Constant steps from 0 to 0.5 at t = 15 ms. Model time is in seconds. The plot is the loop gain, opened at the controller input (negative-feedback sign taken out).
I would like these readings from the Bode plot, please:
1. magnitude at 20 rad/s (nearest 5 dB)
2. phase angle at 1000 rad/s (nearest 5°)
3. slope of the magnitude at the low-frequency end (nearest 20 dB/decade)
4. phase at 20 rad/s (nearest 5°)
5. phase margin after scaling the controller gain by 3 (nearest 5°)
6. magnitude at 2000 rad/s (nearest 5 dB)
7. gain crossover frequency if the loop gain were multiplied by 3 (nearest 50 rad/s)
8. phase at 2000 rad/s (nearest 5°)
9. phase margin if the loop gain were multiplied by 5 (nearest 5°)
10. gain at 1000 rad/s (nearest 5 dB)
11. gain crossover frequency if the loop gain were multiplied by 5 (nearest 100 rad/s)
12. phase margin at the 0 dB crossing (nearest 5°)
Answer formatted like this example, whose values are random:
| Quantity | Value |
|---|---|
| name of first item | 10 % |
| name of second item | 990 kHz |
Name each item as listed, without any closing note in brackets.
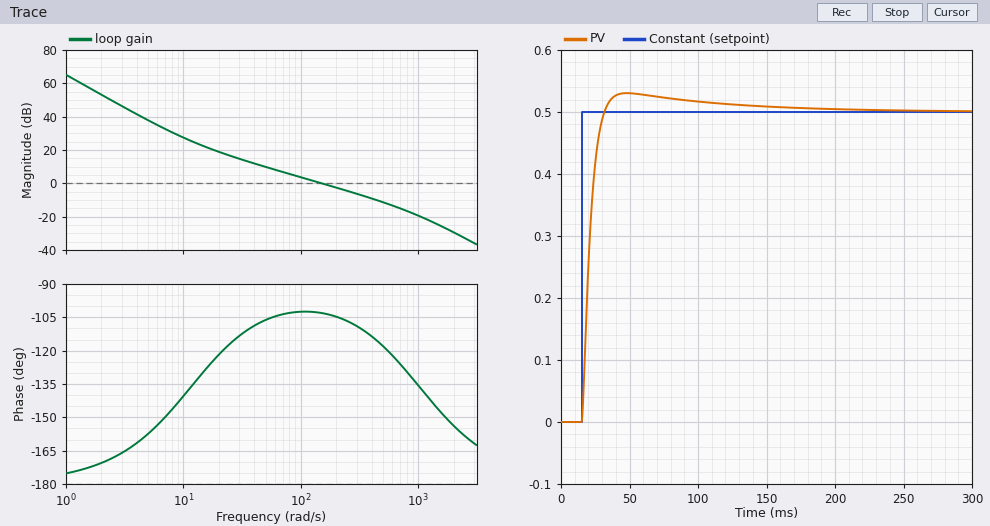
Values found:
| Quantity | Value |
|---|---|
| magnitude at 20 rad/s | 20 dB |
| phase angle at 1000 rad/s | -135° |
| slope of the magnitude at the low-frequency end | -40 dB/decade |
| phase at 20 rad/s | -120° |
| phase margin after scaling the controller gain by 3 | 65° |
| magnitude at 2000 rad/s | -30 dB |
| gain crossover frequency if the loop gain were multiplied by 3 | 400 rad/s |
| phase at 2000 rad/s | -155° |
| phase margin if the loop gain were multiplied by 5 | 55° |
| gain at 1000 rad/s | -20 dB |
| gain crossover frequency if the loop gain were multiplied by 5 | 600 rad/s |
| phase margin at the 0 dB crossing | 75° |
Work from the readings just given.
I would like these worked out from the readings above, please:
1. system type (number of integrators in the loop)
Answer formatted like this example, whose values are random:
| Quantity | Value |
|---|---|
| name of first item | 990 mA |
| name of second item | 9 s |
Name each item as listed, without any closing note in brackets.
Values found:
| Quantity | Value |
|---|---|
| system type | 2 |
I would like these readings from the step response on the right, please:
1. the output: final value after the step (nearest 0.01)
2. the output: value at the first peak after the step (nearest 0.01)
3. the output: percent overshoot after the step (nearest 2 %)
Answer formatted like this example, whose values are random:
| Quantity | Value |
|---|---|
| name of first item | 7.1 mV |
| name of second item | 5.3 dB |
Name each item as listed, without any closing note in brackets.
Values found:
| Quantity | Value |
|---|---|
| the output: final value after the step | 0.50 |
| the output: value at the first peak after the step | 0.53 |
| the output: percent overshoot after the step | 6 % |
